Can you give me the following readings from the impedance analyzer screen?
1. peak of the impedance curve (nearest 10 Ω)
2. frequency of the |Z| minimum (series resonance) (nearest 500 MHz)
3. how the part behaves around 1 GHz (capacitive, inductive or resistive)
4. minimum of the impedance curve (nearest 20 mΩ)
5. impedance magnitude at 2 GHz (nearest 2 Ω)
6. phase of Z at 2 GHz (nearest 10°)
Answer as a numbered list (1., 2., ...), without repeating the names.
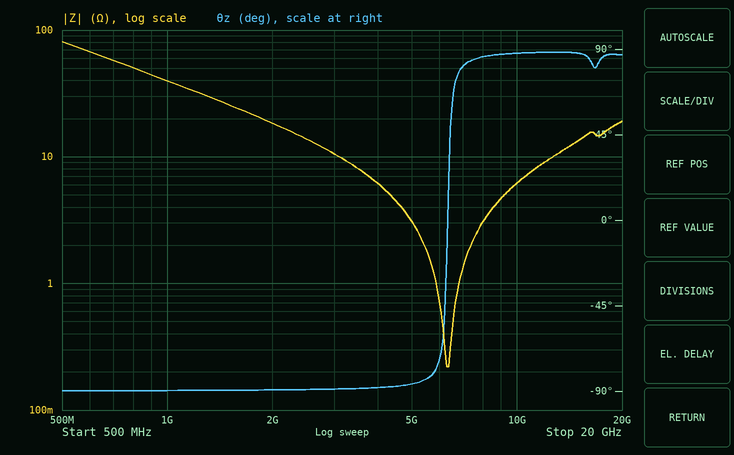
1. 80 Ω
2. 6.5 GHz
3. capacitive
4. 220 mΩ
5. 18 Ω
6. -90°
